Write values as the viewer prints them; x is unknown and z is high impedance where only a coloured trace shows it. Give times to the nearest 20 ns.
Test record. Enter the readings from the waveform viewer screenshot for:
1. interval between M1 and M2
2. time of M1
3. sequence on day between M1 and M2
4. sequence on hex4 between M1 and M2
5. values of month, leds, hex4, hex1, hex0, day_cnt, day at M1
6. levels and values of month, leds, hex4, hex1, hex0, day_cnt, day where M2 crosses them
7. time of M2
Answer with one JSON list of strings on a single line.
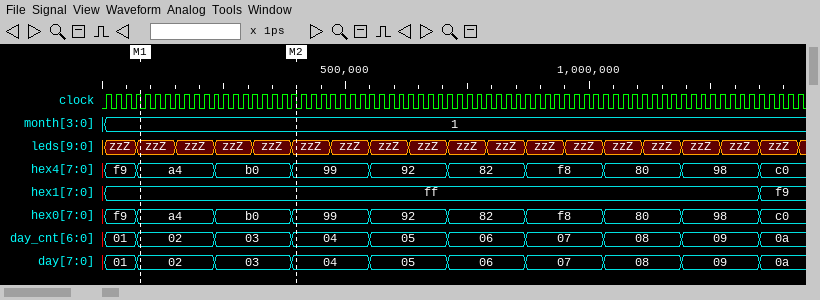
["320 ns", "80 ns", "02, 03, 04", "a4, b0, 99", "month=1, leds=zzZ, hex4=a4, hex1=ff, hex0=a4, day_cnt=02, day=02", "month=1, leds=zzZ, hex4=99, hex1=ff, hex0=99, day_cnt=04, day=04", "400 ns"]
